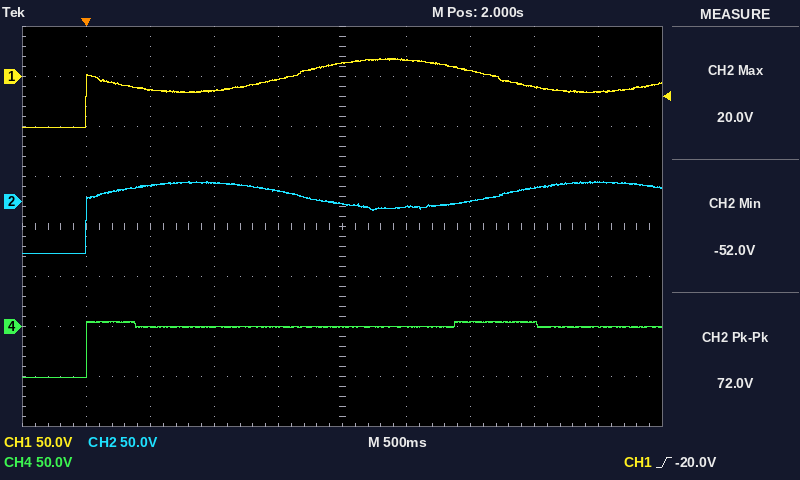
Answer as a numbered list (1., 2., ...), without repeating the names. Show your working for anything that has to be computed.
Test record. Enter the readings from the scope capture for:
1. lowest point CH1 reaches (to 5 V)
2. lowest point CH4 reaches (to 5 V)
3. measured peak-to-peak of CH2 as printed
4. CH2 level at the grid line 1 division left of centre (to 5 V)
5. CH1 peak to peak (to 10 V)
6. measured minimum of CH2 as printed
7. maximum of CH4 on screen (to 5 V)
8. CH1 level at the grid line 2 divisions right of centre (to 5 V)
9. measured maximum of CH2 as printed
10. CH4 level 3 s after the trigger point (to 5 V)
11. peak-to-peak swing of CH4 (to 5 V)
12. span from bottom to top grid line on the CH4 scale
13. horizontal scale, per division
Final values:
1. -50 V
2. -50 V
3. 72.0 V
4. 10 V
5. 70 V
6. -52.0 V
7. 5 V
8. 5 V
9. 20.0 V
10. 5 V
11. 5 V − (-50 V) = 55 V
12. 400 V
13. 500 ms
